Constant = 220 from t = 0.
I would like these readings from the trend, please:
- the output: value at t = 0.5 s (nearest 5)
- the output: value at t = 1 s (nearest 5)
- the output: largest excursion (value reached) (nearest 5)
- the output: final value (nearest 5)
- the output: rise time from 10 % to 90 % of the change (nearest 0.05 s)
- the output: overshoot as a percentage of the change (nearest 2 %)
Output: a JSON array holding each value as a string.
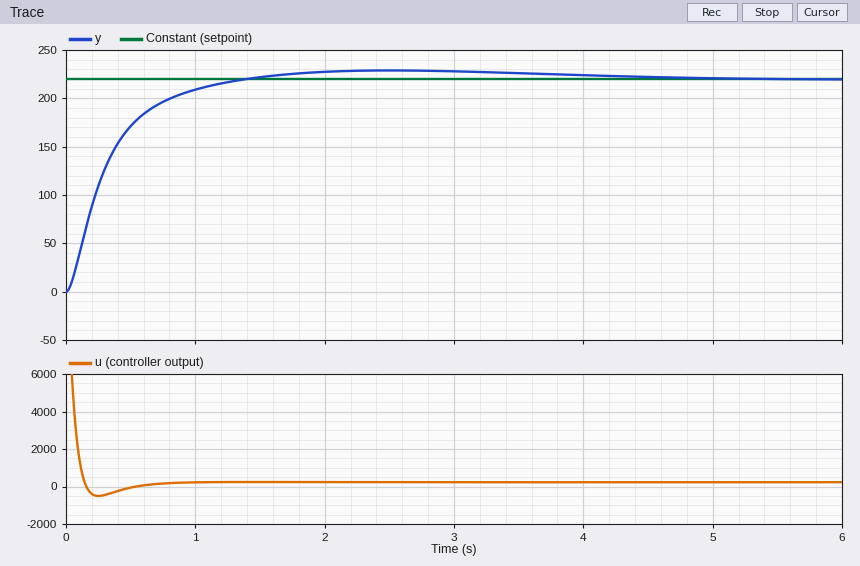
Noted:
["170", "210", "230", "220", "0.70 s", "4 %"]
